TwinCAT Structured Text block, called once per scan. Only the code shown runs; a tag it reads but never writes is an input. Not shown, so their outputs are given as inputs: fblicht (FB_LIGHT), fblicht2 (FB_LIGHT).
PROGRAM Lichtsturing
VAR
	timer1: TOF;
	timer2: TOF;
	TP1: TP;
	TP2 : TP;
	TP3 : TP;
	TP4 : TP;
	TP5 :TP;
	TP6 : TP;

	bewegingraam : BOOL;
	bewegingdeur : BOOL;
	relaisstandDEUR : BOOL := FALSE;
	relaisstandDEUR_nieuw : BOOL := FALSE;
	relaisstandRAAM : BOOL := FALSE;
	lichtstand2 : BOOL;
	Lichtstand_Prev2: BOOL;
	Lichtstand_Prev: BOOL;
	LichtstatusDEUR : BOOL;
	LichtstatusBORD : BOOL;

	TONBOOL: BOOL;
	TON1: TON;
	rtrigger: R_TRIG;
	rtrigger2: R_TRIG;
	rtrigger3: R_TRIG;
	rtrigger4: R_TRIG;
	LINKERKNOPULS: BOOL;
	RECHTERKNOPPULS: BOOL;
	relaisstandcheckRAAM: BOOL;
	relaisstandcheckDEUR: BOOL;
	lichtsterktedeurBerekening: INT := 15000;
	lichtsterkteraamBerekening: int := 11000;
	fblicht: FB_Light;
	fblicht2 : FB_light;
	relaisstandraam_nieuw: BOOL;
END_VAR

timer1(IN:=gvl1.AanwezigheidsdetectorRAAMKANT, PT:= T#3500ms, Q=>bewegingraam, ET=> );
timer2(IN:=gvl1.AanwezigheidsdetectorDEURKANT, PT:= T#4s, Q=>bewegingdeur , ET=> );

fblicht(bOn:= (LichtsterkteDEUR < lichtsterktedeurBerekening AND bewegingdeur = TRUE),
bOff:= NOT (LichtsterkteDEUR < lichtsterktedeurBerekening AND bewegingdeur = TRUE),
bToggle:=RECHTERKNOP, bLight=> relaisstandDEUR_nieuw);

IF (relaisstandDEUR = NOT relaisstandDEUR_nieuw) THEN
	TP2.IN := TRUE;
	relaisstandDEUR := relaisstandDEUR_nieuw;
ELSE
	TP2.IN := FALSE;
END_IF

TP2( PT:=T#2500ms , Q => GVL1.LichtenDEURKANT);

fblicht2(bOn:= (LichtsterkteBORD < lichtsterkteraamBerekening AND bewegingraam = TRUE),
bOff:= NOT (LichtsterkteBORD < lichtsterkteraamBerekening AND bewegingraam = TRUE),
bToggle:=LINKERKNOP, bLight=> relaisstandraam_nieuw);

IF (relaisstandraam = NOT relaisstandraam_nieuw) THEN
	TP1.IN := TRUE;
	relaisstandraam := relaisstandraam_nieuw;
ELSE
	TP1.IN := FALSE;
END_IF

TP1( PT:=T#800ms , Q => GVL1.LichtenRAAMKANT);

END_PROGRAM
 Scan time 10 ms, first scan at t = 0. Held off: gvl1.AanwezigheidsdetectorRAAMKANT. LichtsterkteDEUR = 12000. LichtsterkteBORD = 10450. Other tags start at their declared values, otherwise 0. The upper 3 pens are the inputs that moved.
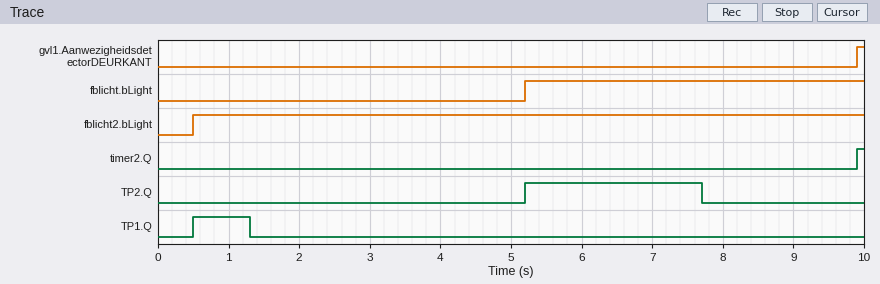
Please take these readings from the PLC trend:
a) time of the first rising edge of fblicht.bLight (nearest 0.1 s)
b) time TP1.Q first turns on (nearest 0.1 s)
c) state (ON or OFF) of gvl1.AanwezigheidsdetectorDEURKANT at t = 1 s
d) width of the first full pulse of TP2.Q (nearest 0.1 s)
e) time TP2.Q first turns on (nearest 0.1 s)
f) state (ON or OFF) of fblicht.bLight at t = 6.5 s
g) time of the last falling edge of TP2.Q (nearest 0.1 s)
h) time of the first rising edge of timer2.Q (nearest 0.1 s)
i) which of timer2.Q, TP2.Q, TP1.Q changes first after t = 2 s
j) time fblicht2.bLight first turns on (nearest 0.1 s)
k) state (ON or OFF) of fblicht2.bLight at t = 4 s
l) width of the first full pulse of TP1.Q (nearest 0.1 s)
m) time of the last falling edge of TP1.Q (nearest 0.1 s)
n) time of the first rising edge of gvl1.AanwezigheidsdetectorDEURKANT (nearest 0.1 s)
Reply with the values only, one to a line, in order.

5.2 s
0.5 s
OFF
2.5 s
5.2 s
ON
7.7 s
9.9 s
TP2.Q
0.5 s
ON
0.8 s
1.3 s
9.9 s
